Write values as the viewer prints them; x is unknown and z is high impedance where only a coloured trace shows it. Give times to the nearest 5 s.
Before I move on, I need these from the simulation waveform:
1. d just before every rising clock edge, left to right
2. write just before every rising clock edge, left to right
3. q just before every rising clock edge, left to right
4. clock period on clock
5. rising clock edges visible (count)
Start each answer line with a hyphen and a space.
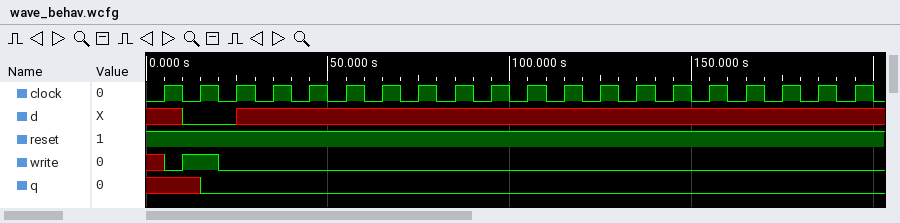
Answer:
- x 0 0 x x x x x x x x x x x x x x x x x
- x 1 0 0 0 0 0 0 0 0 0 0 0 0 0 0 0 0 0 0
- x x 0 0 0 0 0 0 0 0 0 0 0 0 0 0 0 0 0 0
- 10 s
- 20
